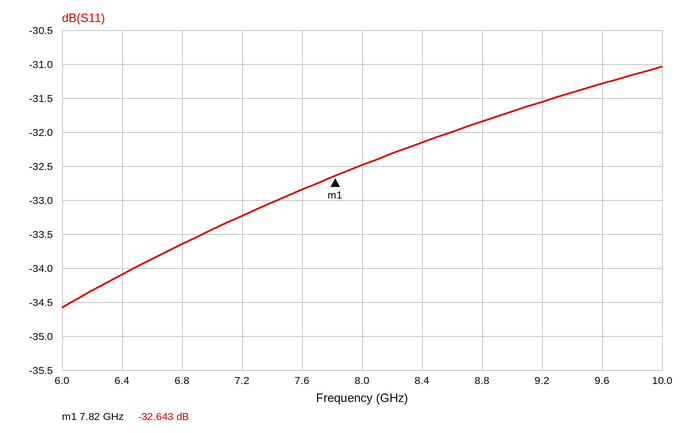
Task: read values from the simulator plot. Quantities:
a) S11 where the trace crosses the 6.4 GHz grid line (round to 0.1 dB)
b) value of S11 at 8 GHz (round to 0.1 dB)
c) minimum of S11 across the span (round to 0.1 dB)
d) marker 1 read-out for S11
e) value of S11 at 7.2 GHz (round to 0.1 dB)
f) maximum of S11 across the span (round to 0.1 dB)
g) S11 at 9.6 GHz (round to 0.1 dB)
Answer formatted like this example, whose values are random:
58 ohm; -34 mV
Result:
-34.1 dB; -32.5 dB; -34.6 dB; -32.643 dB; -33.2 dB; -31.0 dB; -31.3 dB
